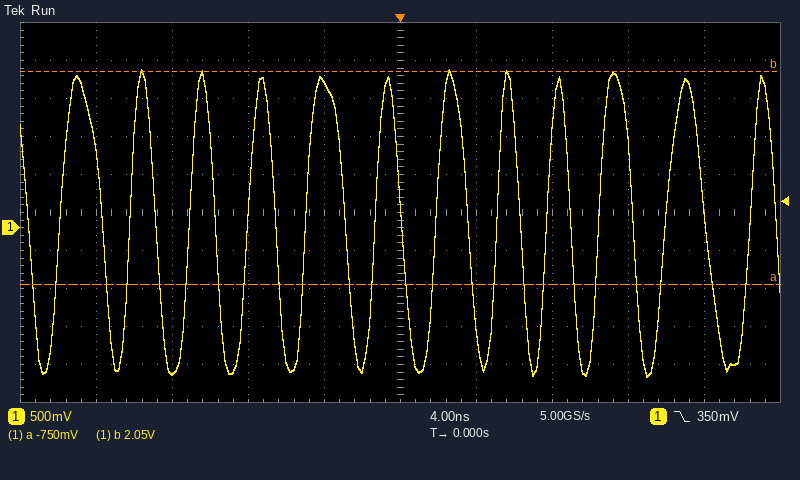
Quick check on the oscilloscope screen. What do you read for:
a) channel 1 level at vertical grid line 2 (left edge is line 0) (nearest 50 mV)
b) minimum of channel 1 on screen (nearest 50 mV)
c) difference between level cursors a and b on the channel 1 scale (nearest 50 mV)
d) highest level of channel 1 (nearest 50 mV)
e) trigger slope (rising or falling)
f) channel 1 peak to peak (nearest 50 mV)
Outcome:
-1.90 V
-1.95 V
2.80 V
2.10 V
falling
4.05 V
